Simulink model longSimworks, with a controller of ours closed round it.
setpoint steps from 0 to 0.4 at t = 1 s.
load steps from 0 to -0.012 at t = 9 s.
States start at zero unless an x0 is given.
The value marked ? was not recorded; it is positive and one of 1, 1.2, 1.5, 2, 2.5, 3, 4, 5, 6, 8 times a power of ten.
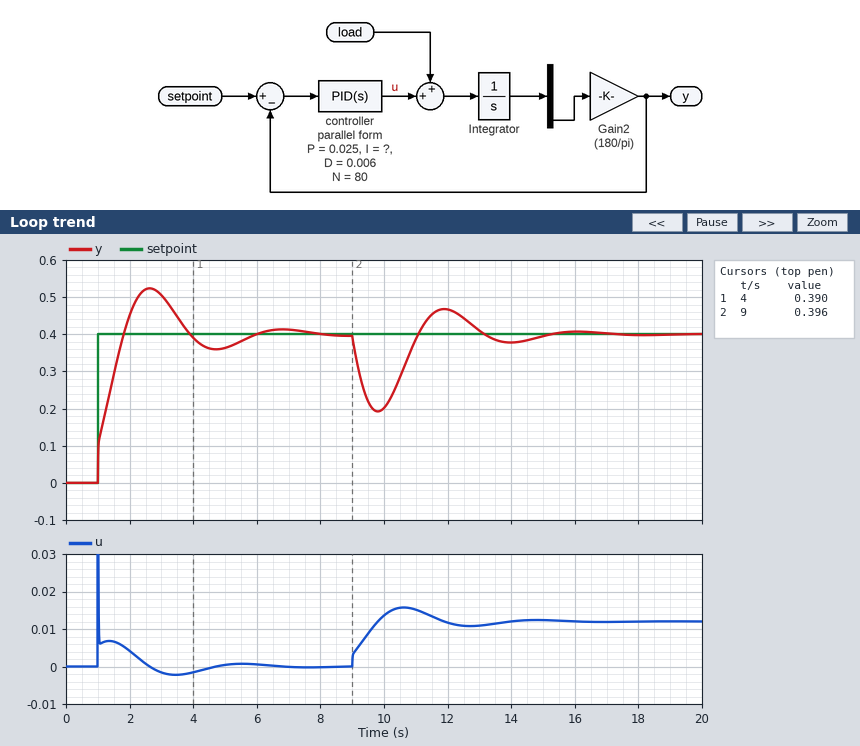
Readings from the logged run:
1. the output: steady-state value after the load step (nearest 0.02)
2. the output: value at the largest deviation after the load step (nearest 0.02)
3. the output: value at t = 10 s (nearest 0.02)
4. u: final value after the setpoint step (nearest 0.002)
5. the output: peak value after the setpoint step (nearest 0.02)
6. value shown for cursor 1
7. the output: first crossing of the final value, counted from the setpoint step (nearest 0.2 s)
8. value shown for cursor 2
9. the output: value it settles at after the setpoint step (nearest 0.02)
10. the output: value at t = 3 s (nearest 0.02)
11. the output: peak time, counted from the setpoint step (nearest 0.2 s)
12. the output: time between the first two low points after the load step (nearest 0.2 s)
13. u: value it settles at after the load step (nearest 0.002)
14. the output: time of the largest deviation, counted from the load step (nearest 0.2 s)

0.40
0.20
0.20
0.000
0.52
0.390
0.8 s
0.396
0.40
0.50
1.6 s
4.2 s
0.012
0.8 s
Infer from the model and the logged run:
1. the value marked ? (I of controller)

0.06
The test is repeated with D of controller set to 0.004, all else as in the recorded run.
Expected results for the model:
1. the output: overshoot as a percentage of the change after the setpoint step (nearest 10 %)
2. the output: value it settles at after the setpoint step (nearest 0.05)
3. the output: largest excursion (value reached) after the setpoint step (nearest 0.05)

30 %
0.40
0.55
